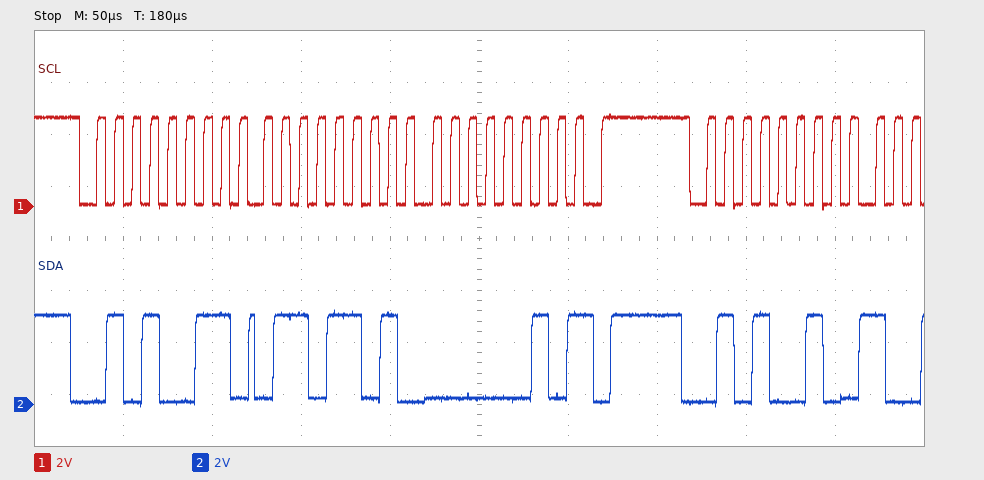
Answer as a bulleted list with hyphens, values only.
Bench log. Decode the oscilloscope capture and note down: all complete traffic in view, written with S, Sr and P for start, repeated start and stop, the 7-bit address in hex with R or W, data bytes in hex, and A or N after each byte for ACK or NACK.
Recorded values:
- S 29R A 6D A 02 N P S 29W A
